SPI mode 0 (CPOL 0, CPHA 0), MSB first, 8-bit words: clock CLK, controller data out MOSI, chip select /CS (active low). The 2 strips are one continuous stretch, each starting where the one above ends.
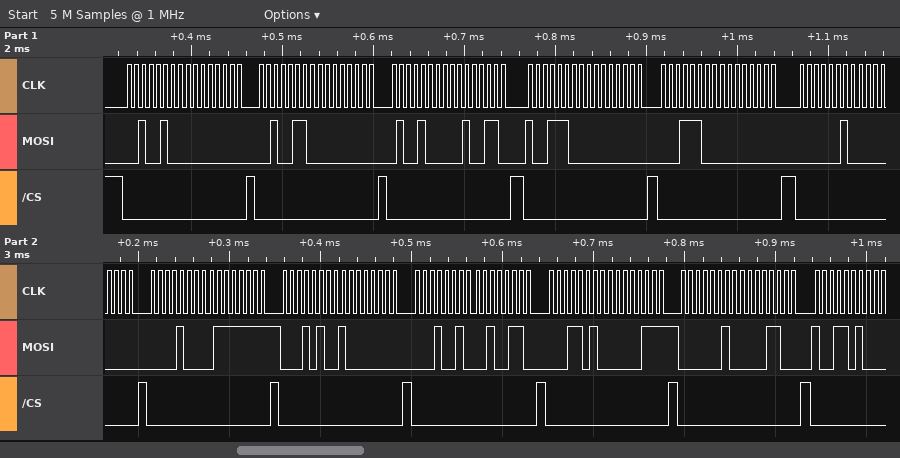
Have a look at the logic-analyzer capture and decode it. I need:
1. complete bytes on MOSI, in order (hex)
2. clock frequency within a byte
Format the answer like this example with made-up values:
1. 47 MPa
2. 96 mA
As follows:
1. 24 00 26 00 48 26 9C 00 1C 00 02 00 08 7F 14 80 12 26 1A 07 02 0C 9A
2. 125 kHz
